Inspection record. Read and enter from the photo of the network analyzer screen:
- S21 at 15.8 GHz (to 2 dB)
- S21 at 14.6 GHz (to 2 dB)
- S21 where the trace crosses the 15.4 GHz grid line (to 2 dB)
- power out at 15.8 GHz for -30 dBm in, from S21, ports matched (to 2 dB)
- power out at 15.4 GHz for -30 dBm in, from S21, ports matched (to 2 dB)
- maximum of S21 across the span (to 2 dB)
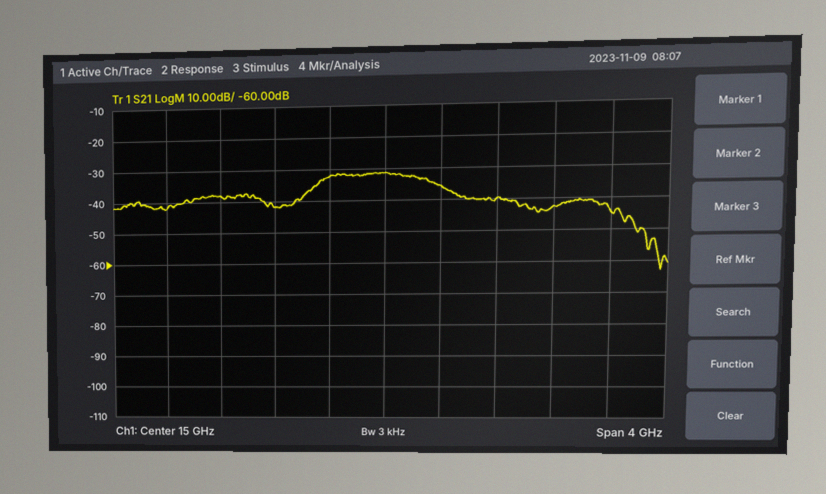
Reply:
-40 dB
-32 dB
-36 dB
-70 dBm
-66 dBm
-32 dB
